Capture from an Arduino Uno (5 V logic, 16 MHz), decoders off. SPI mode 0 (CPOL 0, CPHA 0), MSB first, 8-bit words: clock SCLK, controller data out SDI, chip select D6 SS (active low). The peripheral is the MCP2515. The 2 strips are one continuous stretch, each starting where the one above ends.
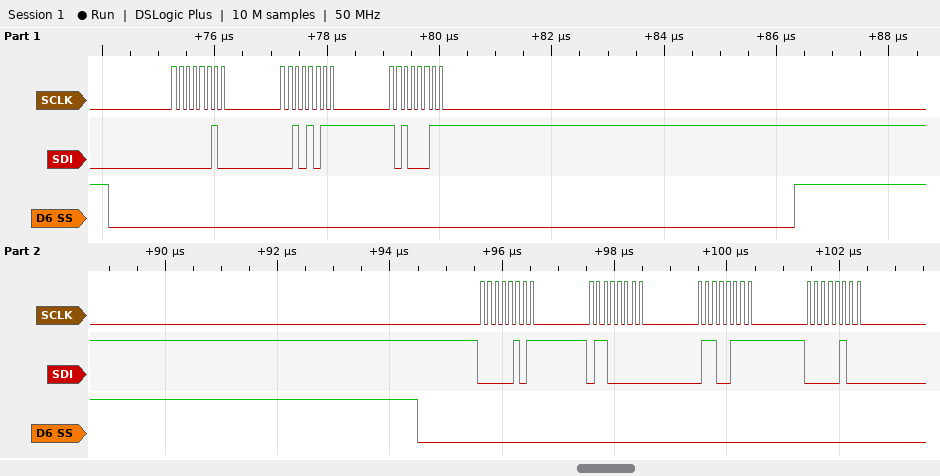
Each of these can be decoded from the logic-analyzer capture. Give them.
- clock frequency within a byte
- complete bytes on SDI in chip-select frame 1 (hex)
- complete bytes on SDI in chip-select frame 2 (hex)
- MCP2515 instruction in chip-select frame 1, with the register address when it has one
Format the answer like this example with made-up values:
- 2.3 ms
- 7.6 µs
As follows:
- 8 MHz
- 02 2B A3
- 05 60 67 04
- WRITE 0x2B
